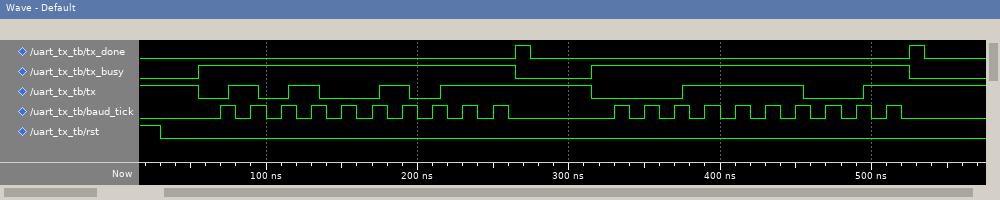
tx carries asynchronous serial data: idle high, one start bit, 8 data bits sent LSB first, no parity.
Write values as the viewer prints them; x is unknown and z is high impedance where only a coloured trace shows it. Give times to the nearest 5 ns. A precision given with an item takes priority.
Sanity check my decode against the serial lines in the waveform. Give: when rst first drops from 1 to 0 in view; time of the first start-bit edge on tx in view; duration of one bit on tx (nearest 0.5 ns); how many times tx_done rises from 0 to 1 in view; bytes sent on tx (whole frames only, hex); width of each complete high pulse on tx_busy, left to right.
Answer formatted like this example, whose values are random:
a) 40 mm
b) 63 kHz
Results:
a) 30 ns
b) 55 ns
c) 20 ns
d) 2
e) A5, 3C
f) 210 ns, 210 ns
